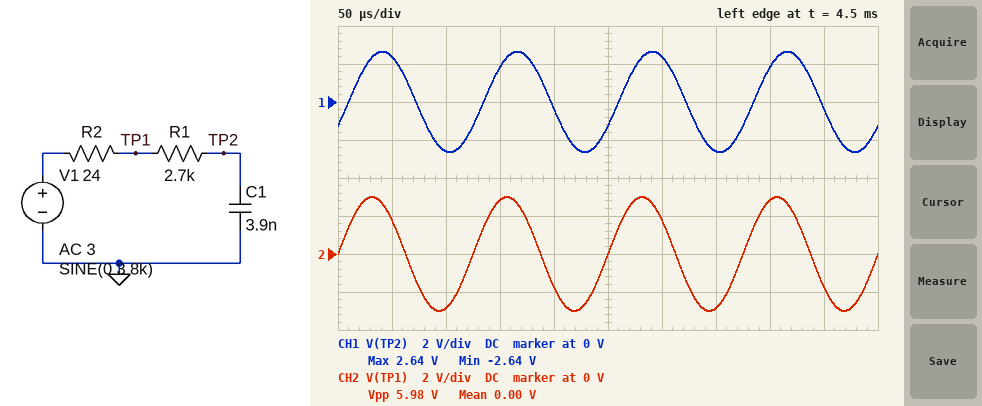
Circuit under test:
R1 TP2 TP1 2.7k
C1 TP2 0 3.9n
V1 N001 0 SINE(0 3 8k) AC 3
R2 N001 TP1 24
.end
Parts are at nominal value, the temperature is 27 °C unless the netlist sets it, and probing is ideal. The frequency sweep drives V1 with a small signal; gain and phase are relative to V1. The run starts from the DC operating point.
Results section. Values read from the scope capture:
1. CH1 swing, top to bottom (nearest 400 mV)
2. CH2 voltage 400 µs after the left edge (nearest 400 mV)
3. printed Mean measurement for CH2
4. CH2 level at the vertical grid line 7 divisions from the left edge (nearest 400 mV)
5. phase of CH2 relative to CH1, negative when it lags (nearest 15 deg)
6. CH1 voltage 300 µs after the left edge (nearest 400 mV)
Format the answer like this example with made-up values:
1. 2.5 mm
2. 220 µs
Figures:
1. 5.2 V
2. 2.8 V
3. 0.00 V
4. -2.8 V
5. 30 deg
6. 2.4 V
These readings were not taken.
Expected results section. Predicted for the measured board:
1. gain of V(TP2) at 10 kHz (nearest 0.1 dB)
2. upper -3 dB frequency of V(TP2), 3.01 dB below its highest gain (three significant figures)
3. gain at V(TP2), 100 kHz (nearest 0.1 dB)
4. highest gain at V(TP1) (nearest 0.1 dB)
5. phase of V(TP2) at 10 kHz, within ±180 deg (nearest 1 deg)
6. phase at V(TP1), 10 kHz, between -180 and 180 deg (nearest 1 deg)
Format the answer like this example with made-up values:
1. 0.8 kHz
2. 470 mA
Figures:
1. -1.6 dB
2. 15.0 kHz
3. -16.6 dB
4. 0 dB
5. -34 deg
6. 0 deg
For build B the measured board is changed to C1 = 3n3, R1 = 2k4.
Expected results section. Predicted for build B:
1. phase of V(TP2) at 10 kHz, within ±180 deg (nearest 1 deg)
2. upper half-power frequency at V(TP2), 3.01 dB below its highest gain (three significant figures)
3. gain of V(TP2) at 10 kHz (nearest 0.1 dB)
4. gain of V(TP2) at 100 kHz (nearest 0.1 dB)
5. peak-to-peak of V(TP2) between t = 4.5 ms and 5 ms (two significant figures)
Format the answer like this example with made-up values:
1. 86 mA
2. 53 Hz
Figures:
1. -27 deg
2. 19.9 kHz
3. -1.0 dB
4. -14.2 dB
5. 5.6 V
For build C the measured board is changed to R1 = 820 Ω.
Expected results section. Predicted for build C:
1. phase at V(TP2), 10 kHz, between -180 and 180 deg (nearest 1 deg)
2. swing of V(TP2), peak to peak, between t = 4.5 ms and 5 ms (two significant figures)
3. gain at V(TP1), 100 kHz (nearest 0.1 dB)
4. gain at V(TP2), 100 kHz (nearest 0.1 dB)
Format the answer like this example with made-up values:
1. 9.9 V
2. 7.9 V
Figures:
1. -12 deg
2. 5.9 V
3. -0.2 dB
4. -7.2 dB
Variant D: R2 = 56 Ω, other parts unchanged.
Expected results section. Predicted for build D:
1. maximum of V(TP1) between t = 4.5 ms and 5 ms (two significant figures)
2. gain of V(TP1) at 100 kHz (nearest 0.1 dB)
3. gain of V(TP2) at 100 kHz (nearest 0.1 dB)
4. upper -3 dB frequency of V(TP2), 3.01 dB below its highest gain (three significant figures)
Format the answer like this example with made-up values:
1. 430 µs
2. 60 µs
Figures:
1. 3.0 V
2. -0.2 dB
3. -16.7 dB
4. 14.8 kHz
